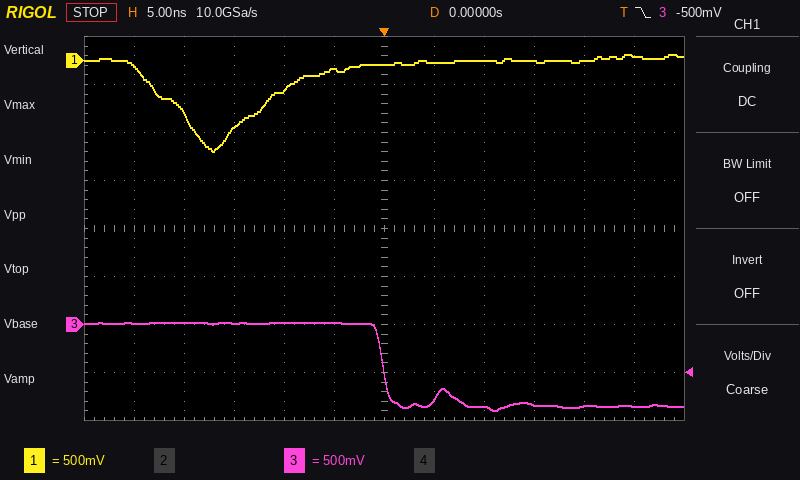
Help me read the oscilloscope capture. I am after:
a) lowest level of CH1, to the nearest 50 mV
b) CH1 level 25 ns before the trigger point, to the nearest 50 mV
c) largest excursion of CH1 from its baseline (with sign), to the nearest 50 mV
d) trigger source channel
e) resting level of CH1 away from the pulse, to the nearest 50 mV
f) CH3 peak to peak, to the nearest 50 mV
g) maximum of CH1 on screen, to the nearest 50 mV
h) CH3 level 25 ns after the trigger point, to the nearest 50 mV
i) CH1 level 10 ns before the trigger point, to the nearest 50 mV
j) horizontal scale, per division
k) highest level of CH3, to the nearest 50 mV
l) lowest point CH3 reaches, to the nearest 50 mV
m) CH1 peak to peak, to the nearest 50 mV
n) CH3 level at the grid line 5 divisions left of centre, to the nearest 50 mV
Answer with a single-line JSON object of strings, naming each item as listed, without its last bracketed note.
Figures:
{"lowest level of CH1, to the nearest 50 mV": "-950 mV", "CH1 level 25 ns before the trigger point, to the nearest 50 mV": "-50 mV", "largest excursion of CH1 from its baseline (with sign), to the nearest 50 mV": "-950 mV", "trigger source channel": "CH3", "resting level of CH1 away from the pulse, to the nearest 50 mV": "0 mV", "CH3 peak to peak, to the nearest 50 mV": "900 mV", "maximum of CH1 on screen, to the nearest 50 mV": "50 mV", "CH3 level 25 ns after the trigger point, to the nearest 50 mV": "-850 mV", "CH1 level 10 ns before the trigger point, to the nearest 50 mV": "-300 mV", "horizontal scale, per division": "5 ns", "highest level of CH3, to the nearest 50 mV": "0 mV", "lowest point CH3 reaches, to the nearest 50 mV": "-900 mV", "CH1 peak to peak, to the nearest 50 mV": "1.00 V", "CH3 level at the grid line 5 divisions left of centre, to the nearest 50 mV": "0 mV"}
